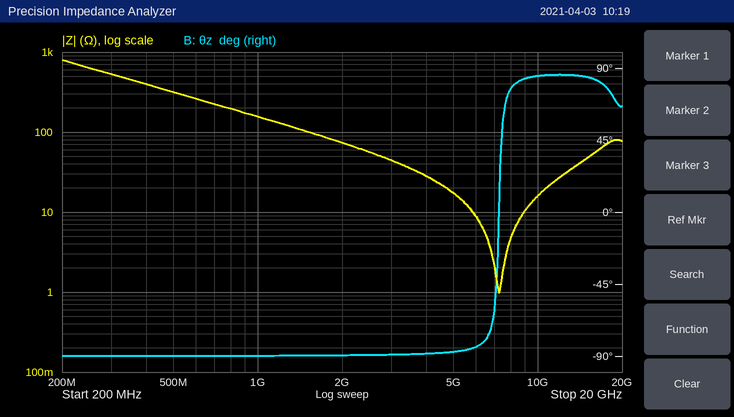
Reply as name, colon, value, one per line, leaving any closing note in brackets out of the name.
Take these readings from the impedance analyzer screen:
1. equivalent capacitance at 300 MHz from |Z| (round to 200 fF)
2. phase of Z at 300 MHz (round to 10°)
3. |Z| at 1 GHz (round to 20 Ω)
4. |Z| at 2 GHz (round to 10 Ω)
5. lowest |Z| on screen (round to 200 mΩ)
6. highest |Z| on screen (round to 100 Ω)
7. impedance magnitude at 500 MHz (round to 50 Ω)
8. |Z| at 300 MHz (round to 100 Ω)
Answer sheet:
equivalent capacitance at 300 MHz from |Z|: 1.0 pF
phase of Z at 300 MHz: -90°
|Z| at 1 GHz: 160 Ω
|Z| at 2 GHz: 70 Ω
lowest |Z| on screen: 1.0 Ω
highest |Z| on screen: 800 Ω
impedance magnitude at 500 MHz: 300 Ω
|Z| at 300 MHz: 500 Ω
